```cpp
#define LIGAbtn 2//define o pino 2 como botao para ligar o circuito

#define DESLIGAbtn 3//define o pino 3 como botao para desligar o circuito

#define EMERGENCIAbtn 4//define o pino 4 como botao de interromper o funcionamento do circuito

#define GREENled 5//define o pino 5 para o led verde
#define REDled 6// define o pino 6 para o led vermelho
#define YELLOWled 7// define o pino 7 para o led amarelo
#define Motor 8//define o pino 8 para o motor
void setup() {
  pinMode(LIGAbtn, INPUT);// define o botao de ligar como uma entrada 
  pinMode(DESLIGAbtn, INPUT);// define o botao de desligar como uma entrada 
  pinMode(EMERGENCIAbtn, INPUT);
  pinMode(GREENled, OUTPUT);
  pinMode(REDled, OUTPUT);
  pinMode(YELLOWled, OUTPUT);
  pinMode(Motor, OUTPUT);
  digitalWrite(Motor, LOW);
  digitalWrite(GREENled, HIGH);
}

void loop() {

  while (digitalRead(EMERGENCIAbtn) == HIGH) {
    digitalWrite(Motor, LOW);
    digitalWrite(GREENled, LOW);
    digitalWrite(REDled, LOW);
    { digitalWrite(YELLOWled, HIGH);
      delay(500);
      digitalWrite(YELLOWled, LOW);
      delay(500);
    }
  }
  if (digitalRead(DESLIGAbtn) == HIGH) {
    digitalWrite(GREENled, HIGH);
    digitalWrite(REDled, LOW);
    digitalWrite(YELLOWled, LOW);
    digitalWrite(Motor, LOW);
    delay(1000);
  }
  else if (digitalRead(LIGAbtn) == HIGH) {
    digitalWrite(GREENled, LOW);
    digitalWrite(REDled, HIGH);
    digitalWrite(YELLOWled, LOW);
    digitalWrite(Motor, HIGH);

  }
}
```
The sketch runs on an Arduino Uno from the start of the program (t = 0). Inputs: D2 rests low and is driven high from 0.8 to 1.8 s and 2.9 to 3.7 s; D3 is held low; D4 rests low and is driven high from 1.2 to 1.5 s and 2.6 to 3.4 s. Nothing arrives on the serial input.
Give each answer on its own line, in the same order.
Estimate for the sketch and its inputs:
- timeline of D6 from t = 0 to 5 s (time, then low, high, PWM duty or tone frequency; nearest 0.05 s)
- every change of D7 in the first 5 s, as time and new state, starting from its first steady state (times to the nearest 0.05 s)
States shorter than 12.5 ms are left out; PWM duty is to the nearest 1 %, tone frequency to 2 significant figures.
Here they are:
0 s low; 0.8 s high; 1.2 s low; 3.6 s high
0 s low; 1.2 s high; 1.7 s low; 2.6 s high; 3.1 s low
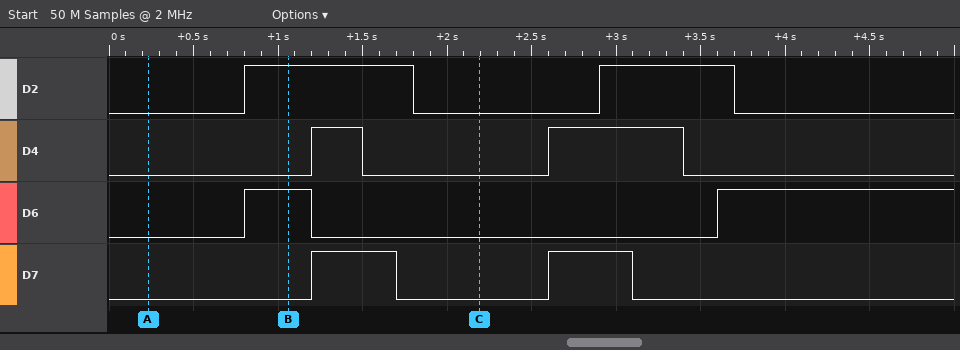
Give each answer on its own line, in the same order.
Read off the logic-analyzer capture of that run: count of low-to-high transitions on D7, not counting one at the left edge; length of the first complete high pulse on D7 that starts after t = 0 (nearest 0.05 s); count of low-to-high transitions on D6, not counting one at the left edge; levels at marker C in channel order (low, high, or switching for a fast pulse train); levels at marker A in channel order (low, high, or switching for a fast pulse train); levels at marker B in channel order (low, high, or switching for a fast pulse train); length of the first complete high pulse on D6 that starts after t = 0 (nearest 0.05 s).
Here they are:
2
0.50 s
2
D2 low, D4 low, D6 low, D7 low
D2 low, D4 low, D6 low, D7 low
D2 high, D4 low, D6 high, D7 low
0.40 s
